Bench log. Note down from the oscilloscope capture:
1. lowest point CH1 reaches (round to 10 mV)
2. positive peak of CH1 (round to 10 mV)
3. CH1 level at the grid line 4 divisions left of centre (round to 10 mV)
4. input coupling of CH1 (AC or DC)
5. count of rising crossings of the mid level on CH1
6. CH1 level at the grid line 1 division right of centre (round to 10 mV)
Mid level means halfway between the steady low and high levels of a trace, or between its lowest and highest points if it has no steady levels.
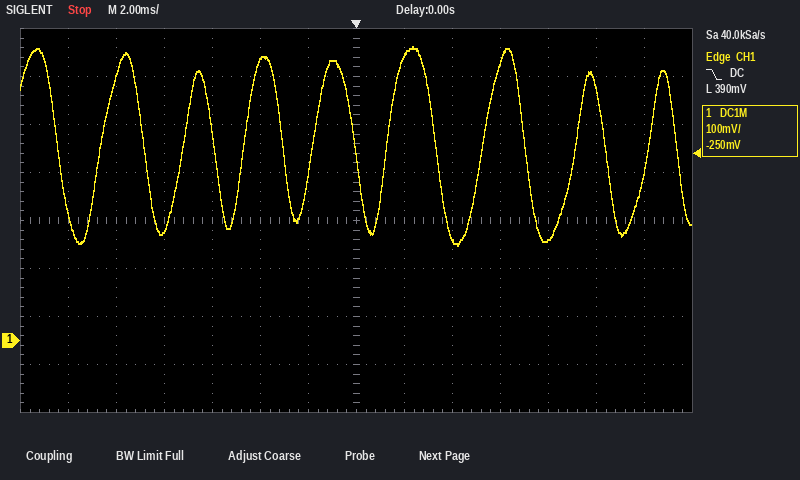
200 mV
610 mV
230 mV
DC
8
590 mV
